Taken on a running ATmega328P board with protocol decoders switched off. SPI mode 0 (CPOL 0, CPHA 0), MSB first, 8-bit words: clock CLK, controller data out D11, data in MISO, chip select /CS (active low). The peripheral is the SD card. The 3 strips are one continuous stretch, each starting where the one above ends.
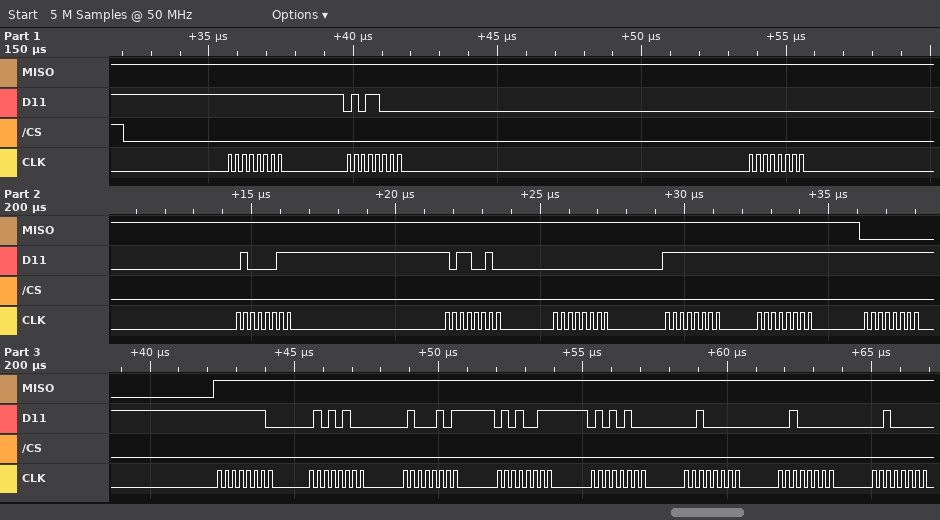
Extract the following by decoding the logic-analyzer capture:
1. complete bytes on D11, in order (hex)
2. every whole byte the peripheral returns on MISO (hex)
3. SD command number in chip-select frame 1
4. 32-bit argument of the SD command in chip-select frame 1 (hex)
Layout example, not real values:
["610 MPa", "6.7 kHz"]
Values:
["FF 58 00 43 B2 00 FF FF FF FE 54 45 53 54 20 20 20", "FF FF FF FF FF FF FF FF 00 FF FF FF FF FF FF FF FF", "CMD24", "0x0043B200"]
